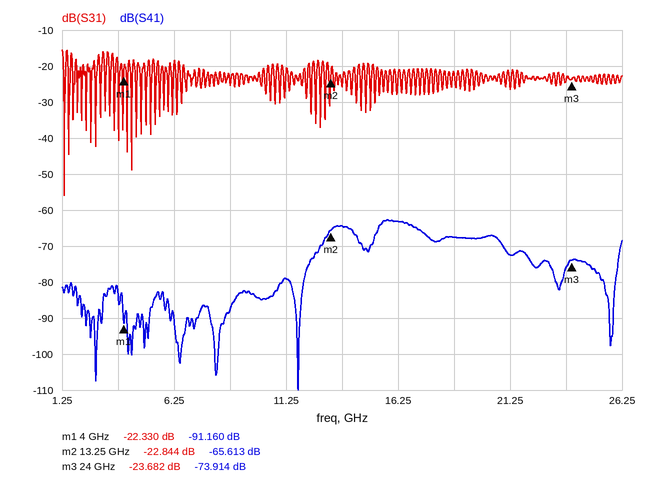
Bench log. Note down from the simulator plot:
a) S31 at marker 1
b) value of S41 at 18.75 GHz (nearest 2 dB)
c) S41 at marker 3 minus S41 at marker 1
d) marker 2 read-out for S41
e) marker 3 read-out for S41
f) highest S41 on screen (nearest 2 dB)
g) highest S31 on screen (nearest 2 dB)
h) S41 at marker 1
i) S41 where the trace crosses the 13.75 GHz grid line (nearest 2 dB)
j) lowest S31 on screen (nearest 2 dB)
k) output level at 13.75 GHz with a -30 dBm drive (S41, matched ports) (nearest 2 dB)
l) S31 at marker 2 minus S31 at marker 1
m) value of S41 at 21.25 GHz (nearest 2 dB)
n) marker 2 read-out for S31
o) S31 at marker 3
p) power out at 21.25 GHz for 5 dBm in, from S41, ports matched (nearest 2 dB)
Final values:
-22.330 dB
-68 dB
17.246 dB
-65.613 dB
-73.914 dB
-62 dB
-16 dB
-91.160 dB
-64 dB
-56 dB
-94 dBm
-0.514 dB
-72 dB
-22.844 dB
-23.682 dB
-68 dBm
